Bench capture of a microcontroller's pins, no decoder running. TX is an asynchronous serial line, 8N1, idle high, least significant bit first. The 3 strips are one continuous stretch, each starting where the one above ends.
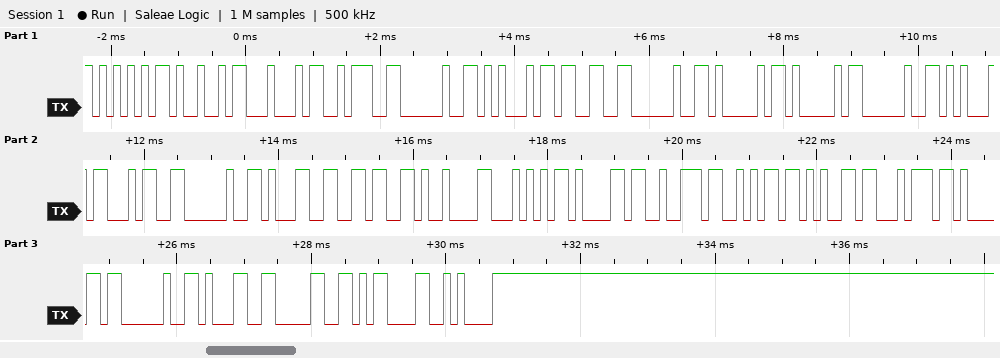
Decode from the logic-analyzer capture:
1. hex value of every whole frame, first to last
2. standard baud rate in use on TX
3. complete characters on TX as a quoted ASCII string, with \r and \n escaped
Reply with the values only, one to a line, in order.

0x55 0x49 0x44 0x3A 0x20 0x45 0x33 0x20 0x41 0x41 0x20 0x45 0x34 0x20 0x31 0x36 0x09 0x54 0x61 0x72 0x6A 0x65 0x74 0x61 0x20 0x31 0x30 0x0D 0x0A
9600 baud
"UID: E3 AA E4 16\tTarjeta 10\r\n"
